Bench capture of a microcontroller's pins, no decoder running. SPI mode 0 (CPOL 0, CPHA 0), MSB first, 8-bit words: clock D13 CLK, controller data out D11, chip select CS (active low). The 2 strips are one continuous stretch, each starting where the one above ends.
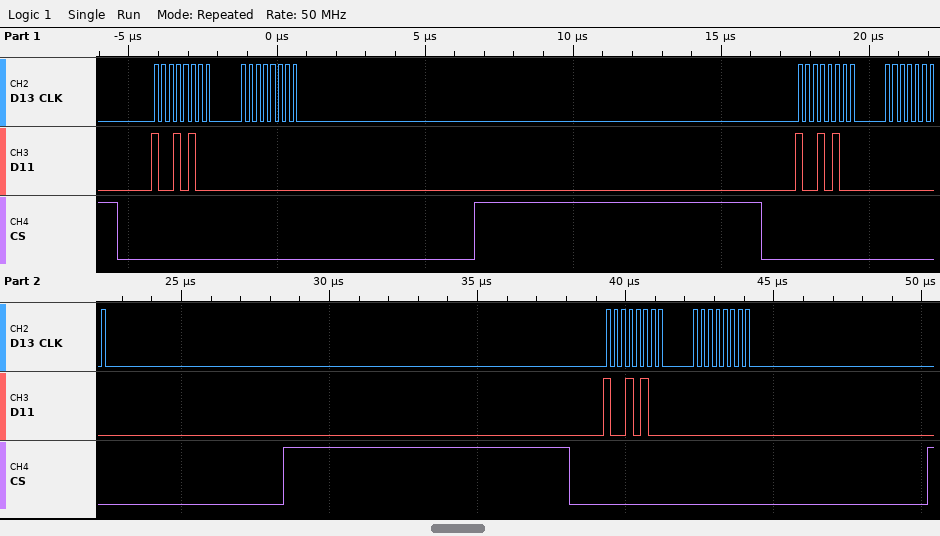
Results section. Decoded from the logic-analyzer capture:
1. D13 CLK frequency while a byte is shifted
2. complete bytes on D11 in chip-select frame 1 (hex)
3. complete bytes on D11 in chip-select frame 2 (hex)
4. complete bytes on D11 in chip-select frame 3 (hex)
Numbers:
4 MHz
94 00
94 00
94 00
